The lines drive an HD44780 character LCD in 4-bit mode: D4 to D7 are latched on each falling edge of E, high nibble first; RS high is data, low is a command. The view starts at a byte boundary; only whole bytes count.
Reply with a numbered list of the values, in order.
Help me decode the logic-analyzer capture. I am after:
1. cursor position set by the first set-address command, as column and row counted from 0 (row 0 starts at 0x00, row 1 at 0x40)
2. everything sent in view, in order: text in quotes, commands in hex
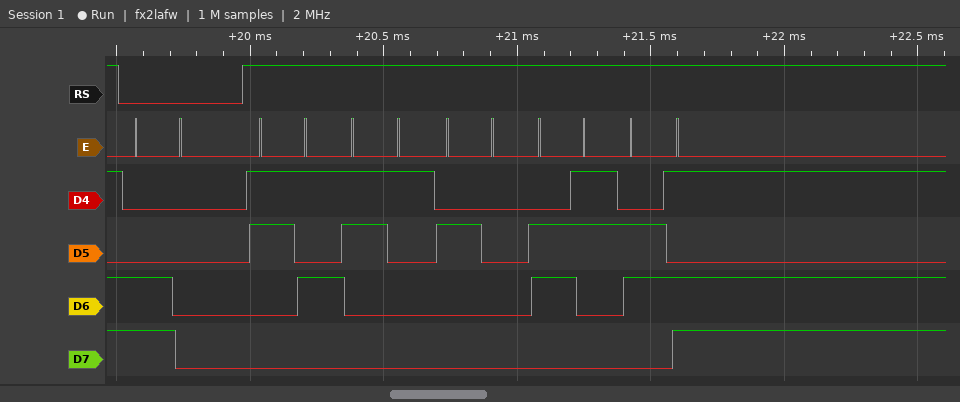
1. column 0, row 1
2. 0xC0 "51 cm"
